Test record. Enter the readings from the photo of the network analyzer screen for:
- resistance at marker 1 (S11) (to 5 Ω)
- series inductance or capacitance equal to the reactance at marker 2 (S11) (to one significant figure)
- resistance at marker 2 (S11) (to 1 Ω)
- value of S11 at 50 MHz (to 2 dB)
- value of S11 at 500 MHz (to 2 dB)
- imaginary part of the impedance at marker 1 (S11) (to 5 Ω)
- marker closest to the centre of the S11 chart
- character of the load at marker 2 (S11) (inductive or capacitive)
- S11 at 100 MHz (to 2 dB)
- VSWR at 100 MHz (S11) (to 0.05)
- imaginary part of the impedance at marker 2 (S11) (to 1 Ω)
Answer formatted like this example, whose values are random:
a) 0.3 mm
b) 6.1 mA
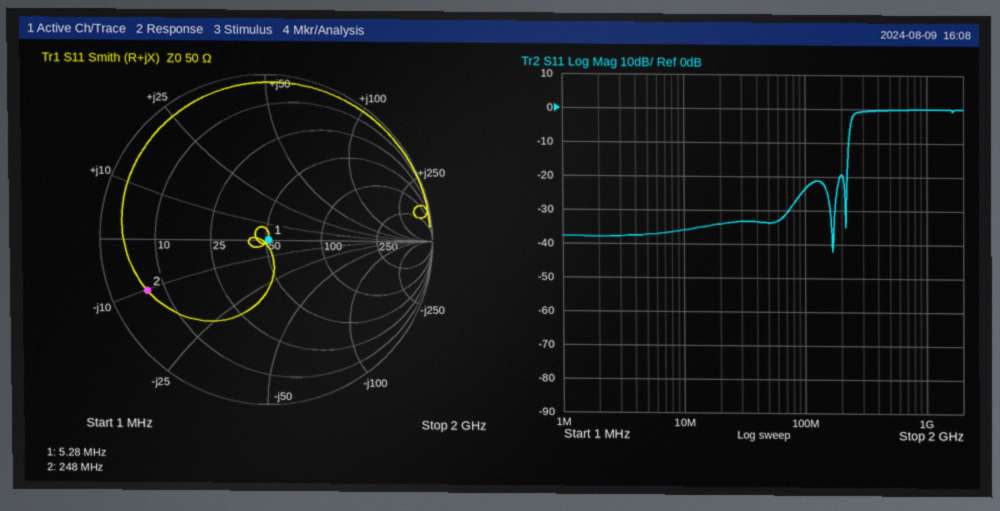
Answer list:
a) 50 Ω
b) 60 pF
c) 6 Ω
d) -34 dB
e) 0 dB
f) 0 Ω
g) marker 1
h) capacitive
i) -24 dB
j) 1.15
k) -10 Ω
